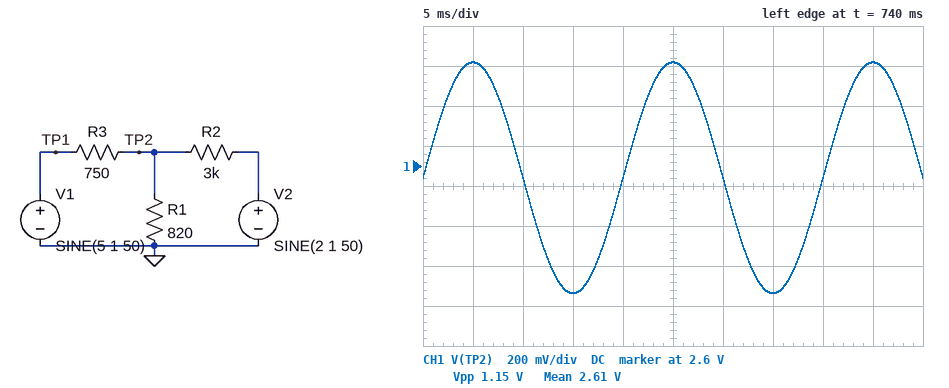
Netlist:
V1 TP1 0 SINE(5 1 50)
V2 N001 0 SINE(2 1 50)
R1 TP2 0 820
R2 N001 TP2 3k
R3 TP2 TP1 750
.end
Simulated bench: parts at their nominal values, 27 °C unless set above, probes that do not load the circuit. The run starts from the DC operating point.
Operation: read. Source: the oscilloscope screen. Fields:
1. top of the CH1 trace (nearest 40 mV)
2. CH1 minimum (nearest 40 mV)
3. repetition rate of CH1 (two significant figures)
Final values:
3.12 V
1.96 V
50 Hz
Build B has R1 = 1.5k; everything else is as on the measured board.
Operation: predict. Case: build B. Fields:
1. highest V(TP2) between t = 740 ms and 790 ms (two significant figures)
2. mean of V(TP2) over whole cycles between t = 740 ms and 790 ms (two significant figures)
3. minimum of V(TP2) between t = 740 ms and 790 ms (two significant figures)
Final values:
3.9 V
3.1 V
2.4 V
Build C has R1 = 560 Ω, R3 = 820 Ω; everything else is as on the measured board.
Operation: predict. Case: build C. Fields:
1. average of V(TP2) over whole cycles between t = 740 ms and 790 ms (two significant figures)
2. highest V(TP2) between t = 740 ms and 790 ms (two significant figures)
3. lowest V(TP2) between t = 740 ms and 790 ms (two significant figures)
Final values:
2.0 V
2.5 V
1.6 V
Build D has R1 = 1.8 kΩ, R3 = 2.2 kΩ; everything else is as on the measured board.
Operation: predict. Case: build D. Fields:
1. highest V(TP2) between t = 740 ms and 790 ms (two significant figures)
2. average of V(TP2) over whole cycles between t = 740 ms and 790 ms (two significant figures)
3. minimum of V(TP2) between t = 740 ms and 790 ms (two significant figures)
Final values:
2.8 V
2.2 V
1.6 V
